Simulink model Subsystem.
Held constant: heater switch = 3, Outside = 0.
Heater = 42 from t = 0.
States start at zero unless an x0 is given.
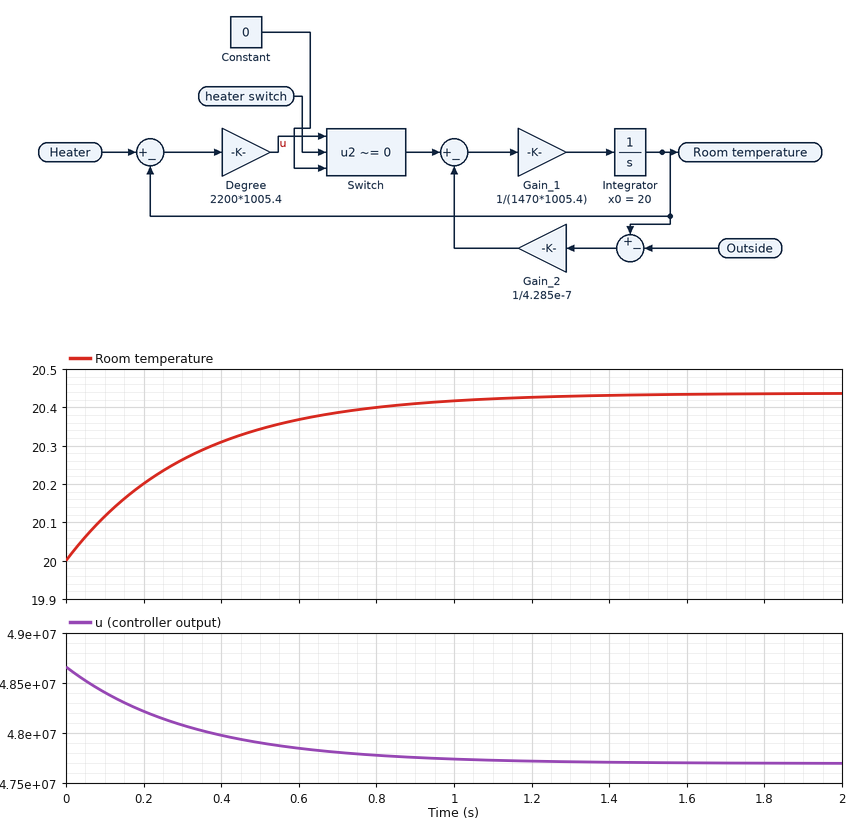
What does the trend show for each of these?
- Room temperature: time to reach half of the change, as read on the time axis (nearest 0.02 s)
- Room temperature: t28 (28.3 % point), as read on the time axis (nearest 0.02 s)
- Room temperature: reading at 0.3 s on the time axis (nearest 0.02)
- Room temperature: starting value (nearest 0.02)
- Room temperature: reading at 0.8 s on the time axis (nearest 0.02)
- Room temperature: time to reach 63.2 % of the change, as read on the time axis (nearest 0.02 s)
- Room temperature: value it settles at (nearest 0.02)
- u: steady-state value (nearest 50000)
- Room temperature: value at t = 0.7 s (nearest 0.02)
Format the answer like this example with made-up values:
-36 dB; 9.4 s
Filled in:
0.22 s; 0.10 s; 20.26; 20.00; 20.40; 0.32 s; 20.44; 47700000; 20.38
